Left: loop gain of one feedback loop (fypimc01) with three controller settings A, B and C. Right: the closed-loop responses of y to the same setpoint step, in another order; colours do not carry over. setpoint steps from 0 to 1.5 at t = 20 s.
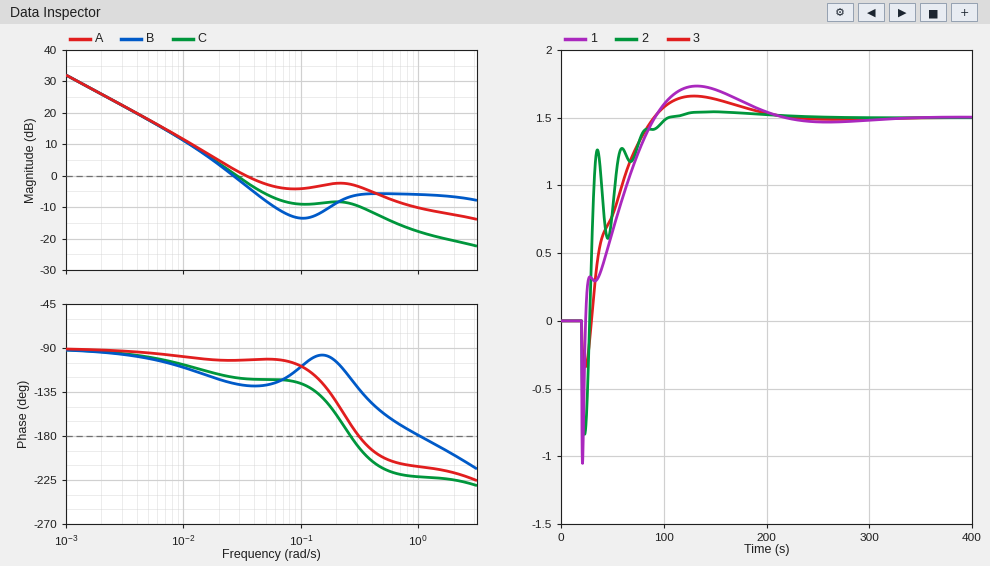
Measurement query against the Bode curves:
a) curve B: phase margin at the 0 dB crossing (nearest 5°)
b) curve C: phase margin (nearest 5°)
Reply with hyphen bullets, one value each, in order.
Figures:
- 55°
- 60°
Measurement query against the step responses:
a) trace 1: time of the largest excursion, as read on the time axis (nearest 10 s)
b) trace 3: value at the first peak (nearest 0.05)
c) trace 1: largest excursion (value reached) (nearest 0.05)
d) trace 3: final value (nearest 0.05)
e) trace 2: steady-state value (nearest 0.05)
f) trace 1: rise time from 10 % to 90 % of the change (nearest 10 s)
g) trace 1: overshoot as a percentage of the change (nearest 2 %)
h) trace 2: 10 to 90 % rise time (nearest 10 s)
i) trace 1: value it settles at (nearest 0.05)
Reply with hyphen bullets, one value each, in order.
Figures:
- 130 s
- 1.65
- 1.75
- 1.50
- 1.50
- 60 s
- 16 %
- 50 s
- 1.50
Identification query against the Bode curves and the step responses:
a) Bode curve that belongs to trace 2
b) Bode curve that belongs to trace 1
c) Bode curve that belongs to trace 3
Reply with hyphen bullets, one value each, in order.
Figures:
- A
- B
- C
